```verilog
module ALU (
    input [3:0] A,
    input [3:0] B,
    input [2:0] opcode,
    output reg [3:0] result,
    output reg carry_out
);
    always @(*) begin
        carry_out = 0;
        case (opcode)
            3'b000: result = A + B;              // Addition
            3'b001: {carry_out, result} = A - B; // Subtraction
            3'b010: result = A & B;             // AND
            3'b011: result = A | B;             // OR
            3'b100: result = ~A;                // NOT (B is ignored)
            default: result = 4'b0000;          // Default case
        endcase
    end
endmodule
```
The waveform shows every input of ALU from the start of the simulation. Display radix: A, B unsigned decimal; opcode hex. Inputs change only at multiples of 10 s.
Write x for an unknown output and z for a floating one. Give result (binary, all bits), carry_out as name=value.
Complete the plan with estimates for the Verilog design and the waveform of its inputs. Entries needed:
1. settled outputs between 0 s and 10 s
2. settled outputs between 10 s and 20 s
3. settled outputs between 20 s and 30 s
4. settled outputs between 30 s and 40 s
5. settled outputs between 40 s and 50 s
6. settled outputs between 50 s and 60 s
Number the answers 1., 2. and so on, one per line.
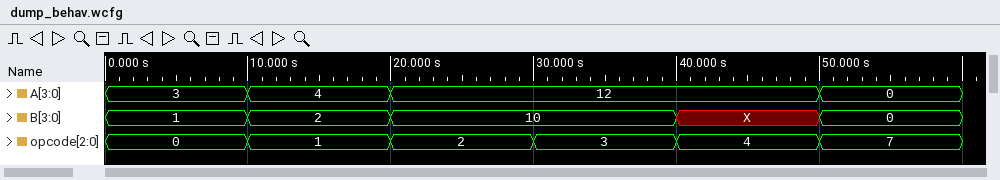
1. result=0100, carry_out=0
2. result=0010, carry_out=0
3. result=1000, carry_out=0
4. result=1110, carry_out=0
5. result=0011, carry_out=0
6. result=0000, carry_out=0
